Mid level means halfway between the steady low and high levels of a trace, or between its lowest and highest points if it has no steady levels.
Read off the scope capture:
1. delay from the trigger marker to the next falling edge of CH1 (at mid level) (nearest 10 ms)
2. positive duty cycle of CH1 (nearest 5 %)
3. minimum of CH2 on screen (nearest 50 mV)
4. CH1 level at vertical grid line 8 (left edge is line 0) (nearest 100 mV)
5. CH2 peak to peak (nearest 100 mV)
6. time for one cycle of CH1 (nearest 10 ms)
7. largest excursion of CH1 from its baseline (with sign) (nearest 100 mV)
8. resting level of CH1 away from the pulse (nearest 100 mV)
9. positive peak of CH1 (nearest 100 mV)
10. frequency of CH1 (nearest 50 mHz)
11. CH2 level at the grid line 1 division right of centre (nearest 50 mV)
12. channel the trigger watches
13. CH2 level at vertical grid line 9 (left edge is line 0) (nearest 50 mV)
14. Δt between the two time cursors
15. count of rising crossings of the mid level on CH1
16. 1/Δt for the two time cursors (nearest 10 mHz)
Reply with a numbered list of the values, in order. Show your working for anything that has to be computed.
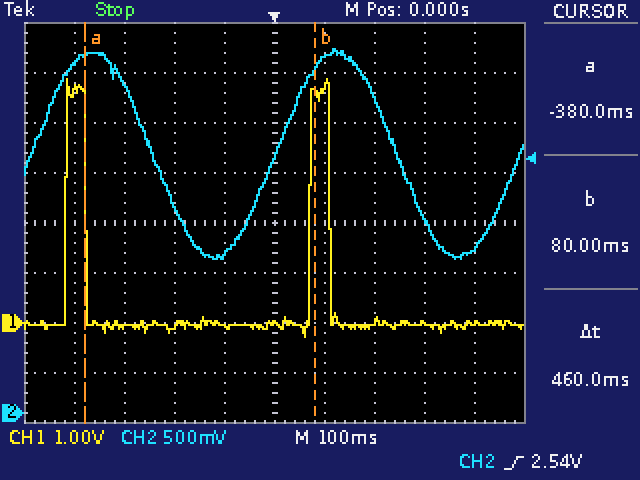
1. 110 ms
2. 10 %
3. 1.55 V
4. 0.0 V
5. 2.10 V
6. 490 ms
7. 4.9 V − (0.0 V) = +4.9 V
8. 0.0 V
9. 4.9 V
10. 1 / 490 ms ≈ 2.04 Hz, so 2.05 Hz to the nearest 50 mHz
11. 3.55 V
12. CH2
13. 1.65 V
14. 460 ms
15. 2
16. 1 / 460 ms ≈ 2.17 Hz
